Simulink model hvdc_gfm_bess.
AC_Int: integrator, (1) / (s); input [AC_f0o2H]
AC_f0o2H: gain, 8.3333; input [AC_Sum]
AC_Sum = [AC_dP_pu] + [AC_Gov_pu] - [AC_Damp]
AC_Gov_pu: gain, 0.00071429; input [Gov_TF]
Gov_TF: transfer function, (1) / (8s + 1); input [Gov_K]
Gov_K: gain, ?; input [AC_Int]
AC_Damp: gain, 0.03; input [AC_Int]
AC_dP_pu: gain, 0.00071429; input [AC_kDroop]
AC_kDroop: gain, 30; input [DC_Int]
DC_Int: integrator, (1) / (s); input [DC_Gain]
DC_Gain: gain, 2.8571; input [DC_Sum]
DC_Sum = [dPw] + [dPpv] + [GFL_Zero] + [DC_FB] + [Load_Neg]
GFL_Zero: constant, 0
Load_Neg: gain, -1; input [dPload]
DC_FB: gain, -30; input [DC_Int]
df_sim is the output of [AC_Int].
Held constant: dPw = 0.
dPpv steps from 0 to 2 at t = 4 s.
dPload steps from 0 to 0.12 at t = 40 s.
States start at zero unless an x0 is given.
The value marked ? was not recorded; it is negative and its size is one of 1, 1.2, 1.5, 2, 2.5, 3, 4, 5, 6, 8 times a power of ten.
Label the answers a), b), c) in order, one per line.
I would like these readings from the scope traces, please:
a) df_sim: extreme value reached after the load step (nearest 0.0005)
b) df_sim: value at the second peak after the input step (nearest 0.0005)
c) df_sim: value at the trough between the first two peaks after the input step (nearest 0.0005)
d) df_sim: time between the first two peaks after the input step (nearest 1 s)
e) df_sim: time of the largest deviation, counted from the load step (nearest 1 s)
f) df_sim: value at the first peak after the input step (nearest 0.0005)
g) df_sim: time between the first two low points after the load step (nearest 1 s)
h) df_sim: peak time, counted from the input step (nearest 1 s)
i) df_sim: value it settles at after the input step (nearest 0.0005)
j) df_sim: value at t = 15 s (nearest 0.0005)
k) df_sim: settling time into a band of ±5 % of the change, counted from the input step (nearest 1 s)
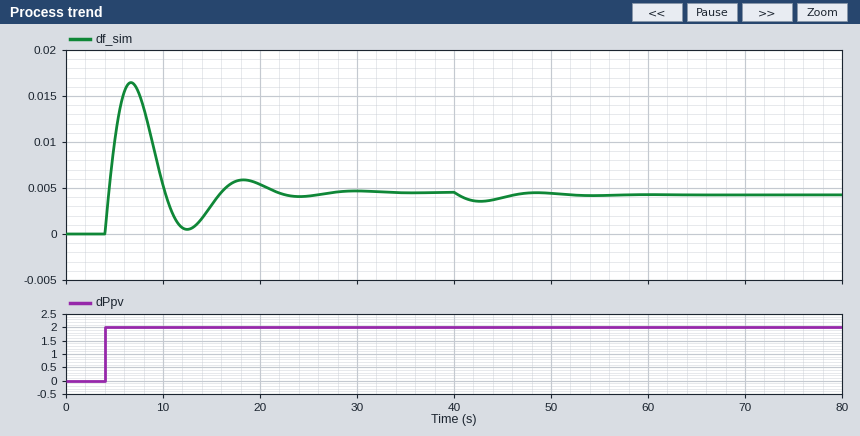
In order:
a) 0.0035
b) 0.0060
c) 0.0005
d) 12 s
e) 3 s
f) 0.0165
g) 12 s
h) 3 s
i) 0.0045
j) 0.0030
k) 22 s
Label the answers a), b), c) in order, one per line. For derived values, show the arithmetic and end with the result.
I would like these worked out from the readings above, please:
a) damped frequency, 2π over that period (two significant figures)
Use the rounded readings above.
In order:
a) 2π / 12 = 0.52 rad/s
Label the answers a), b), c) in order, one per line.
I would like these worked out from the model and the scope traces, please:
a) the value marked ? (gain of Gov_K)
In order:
a) -400
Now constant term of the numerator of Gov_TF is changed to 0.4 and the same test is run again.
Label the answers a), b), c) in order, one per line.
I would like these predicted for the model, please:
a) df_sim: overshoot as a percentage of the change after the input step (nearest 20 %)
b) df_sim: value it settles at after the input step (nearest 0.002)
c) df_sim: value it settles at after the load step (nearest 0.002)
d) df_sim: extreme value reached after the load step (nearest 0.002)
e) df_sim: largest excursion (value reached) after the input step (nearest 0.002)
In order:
a) 120 %
b) 0.010
c) 0.010
d) 0.008
e) 0.022
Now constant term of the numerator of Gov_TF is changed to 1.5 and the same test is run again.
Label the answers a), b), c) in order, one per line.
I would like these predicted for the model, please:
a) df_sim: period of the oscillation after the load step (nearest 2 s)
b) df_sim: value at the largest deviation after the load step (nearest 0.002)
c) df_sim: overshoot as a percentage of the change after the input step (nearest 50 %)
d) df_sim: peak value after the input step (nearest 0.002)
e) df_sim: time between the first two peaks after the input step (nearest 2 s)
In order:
a) 10 s
b) 0.002
c) 350 %
d) 0.014
e) 10 s
